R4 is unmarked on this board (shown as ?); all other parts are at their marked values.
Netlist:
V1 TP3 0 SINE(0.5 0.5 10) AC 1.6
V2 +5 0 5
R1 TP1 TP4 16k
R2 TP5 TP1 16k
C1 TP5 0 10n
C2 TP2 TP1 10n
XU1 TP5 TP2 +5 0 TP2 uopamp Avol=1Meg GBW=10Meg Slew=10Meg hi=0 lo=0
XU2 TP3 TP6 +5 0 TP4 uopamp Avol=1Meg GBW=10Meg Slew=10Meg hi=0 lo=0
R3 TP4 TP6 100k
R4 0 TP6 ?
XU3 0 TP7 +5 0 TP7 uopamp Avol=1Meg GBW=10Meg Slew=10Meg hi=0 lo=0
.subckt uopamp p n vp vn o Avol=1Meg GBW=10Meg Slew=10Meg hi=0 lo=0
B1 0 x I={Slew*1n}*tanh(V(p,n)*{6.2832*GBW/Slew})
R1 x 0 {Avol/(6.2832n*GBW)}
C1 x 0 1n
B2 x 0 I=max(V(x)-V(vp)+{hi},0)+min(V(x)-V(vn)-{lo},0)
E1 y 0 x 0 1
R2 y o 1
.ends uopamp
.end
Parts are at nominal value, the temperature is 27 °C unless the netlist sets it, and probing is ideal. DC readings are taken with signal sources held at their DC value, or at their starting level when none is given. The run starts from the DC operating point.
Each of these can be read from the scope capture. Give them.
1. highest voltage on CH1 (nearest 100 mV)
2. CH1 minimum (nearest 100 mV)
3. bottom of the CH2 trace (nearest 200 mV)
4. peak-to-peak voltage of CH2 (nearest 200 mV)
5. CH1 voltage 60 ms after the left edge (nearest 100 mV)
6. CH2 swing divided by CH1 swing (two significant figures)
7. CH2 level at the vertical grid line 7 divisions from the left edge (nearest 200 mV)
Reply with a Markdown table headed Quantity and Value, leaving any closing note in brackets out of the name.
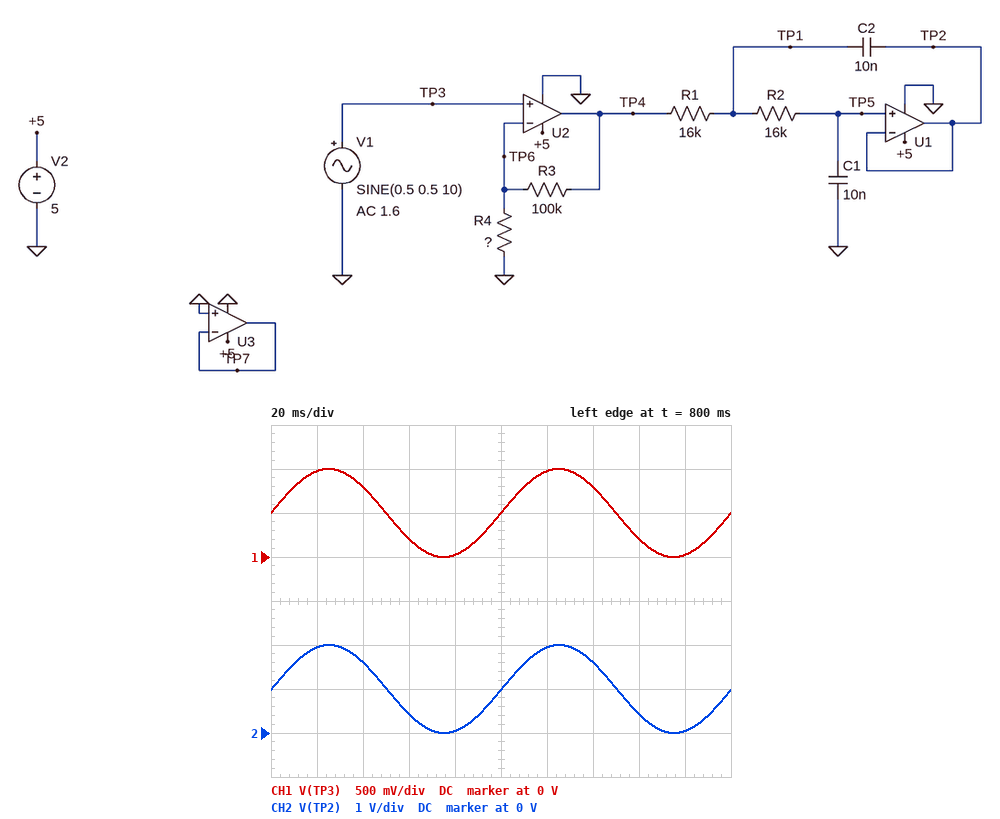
| Quantity | Value |
|---|---|
| highest voltage on CH1 | 1.0 V |
| CH1 minimum | 0 V |
| bottom of the CH2 trace | 0 V |
| peak-to-peak voltage of CH2 | 2.0 V |
| CH1 voltage 60 ms after the left edge | 200 mV |
| CH2 swing divided by CH1 swing | 2.0 |
| CH2 level at the vertical grid line 7 divisions from the left edge | 1.6 V |
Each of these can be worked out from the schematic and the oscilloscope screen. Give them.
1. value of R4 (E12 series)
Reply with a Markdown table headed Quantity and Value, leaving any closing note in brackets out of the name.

| Quantity | Value |
|---|---|
| value of R4 | 100 kΩ |
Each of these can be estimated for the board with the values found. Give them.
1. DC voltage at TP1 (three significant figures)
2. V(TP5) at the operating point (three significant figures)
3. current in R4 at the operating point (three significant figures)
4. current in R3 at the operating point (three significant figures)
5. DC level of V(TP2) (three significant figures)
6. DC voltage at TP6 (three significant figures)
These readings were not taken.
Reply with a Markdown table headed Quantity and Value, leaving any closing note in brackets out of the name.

| Quantity | Value |
|---|---|
| DC voltage at TP1 | 1.00 V |
| V(TP5) at the operating point | 1.00 V |
| current in R4 at the operating point | 5.00 µA |
| current in R3 at the operating point | 5.00 µA |
| DC level of V(TP2) | 1.00 V |
| DC voltage at TP6 | 500 mV |
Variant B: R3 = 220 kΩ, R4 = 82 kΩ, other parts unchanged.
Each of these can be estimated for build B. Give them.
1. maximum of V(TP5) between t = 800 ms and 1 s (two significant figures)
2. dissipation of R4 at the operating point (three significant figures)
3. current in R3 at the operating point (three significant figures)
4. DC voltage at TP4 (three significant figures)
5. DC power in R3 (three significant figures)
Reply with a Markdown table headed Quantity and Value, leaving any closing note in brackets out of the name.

| Quantity | Value |
|---|---|
| maximum of V(TP5) between t = 800 ms and 1 s | 3.7 V |
| dissipation of R4 at the operating point | 3.05 µW |
| current in R3 at the operating point | 6.10 µA |
| DC voltage at TP4 | 1.84 V |
| DC power in R3 | 8.18 µW |
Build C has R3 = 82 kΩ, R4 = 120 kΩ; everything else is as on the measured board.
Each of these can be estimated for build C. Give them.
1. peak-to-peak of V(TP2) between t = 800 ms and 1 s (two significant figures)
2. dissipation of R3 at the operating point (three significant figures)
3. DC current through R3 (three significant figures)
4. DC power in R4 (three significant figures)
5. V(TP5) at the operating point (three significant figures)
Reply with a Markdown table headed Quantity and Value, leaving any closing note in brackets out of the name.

| Quantity | Value |
|---|---|
| peak-to-peak of V(TP2) between t = 800 ms and 1 s | 1.7 V |
| dissipation of R3 at the operating point | 1.42 µW |
| DC current through R3 | 4.17 µA |
| DC power in R4 | 2.08 µW |
| V(TP5) at the operating point | 842 mV |
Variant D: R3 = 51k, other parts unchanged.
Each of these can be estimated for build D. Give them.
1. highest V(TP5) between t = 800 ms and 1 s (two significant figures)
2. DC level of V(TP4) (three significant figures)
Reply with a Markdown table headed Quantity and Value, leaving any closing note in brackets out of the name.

| Quantity | Value |
|---|---|
| highest V(TP5) between t = 800 ms and 1 s | 1.5 V |
| DC level of V(TP4) | 755 mV |
